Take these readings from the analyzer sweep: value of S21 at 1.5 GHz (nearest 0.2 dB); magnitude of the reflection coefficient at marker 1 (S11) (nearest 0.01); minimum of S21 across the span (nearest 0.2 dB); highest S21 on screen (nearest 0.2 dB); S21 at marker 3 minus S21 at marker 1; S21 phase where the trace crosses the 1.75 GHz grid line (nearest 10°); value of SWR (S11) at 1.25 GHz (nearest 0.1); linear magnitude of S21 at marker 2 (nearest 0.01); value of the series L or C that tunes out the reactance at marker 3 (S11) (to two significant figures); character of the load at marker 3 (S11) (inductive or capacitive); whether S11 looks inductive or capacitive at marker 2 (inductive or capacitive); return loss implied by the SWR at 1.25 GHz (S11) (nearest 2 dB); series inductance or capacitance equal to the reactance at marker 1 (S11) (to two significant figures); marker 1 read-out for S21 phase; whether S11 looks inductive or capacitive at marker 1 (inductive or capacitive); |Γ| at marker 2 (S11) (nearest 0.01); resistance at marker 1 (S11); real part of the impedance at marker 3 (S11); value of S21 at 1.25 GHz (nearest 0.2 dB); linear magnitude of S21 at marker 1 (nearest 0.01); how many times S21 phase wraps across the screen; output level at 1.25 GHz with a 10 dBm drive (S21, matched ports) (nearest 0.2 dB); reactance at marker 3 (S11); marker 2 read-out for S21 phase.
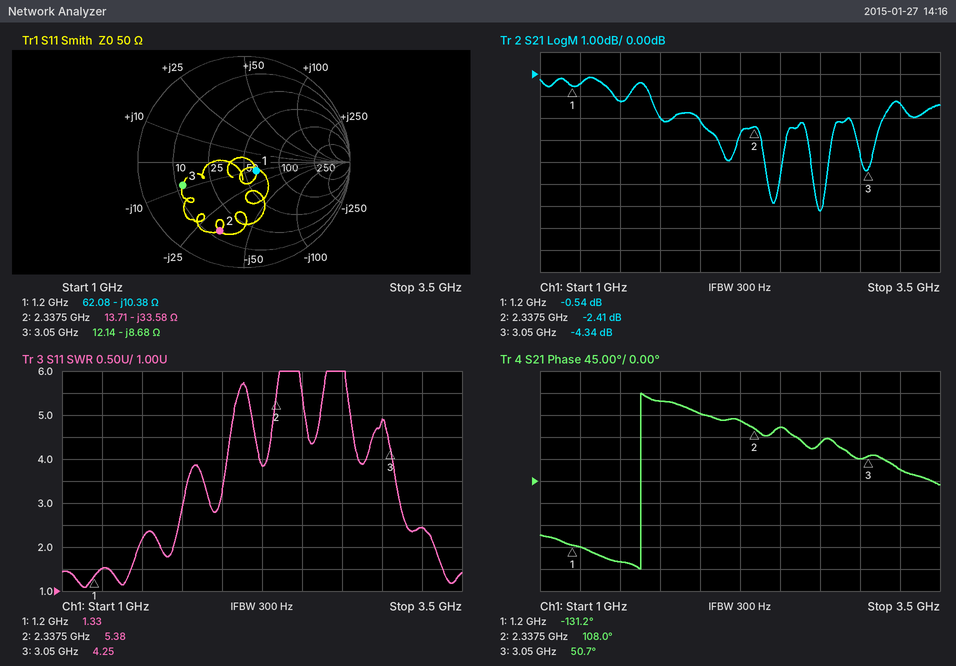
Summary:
-1.2 dB
0.14
-6.2 dB
-0.2 dB
-3.80 dB
160°
1.5
0.76
450 pH
capacitive
capacitive
14 dB
13 pF
-131.2°
capacitive
0.69
62.08 Ω
12.14 Ω
-0.4 dB
0.94
1
9.6 dBm
-8.68 Ω
108.0°
